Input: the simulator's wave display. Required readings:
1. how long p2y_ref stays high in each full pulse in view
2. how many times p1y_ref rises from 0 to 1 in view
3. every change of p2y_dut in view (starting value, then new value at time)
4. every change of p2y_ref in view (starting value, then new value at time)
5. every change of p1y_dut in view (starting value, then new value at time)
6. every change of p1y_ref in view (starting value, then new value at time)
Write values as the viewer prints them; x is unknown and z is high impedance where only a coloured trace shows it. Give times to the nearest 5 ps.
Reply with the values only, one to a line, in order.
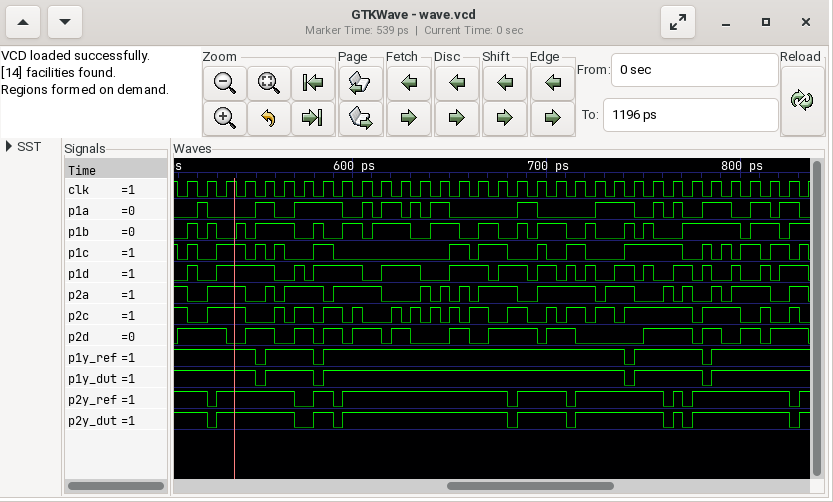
40 ps, 10 ps, 85 ps, 25 ps, 45 ps, 5 ps, 50 ps
4
1, 0 at 525 ps, 1 at 530 ps, 0 at 570 ps, 1 at 580 ps, 0 at 590 ps, 1 at 595 ps, 0 at 680 ps, 1 at 685 ps, 0 at 710 ps, 1 at 715 ps, 0 at 760 ps, 1 at 765 ps, 0 at 770 ps, 1 at 775 ps, 0 at 825 ps, 1 at 830 ps
1, 0 at 525 ps, 1 at 530 ps, 0 at 570 ps, 1 at 580 ps, 0 at 590 ps, 1 at 595 ps, 0 at 680 ps, 1 at 685 ps, 0 at 710 ps, 1 at 715 ps, 0 at 760 ps, 1 at 765 ps, 0 at 770 ps, 1 at 775 ps, 0 at 825 ps, 1 at 830 ps
1, 0 at 550 ps, 1 at 555 ps, 0 at 580 ps, 1 at 585 ps, 0 at 740 ps, 1 at 745 ps, 0 at 780 ps, 1 at 785 ps
1, 0 at 550 ps, 1 at 555 ps, 0 at 580 ps, 1 at 585 ps, 0 at 740 ps, 1 at 745 ps, 0 at 780 ps, 1 at 785 ps
